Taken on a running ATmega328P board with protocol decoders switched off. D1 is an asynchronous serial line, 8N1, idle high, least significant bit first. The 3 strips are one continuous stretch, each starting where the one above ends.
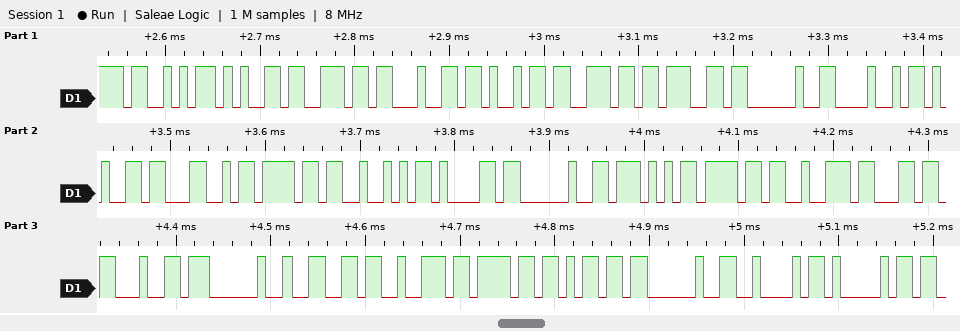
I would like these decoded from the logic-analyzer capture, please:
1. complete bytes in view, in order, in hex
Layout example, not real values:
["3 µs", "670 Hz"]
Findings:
["0x53 0x65 0x6E 0x64 0x69 0x6E 0x67 0x20 0x48 0x65 0x4C 0x6F 0x52 0x61 0x20 0x57 0x6F 0x72 0x6C 0x64 0x20 0x66 0x72 0x6F 0x6D 0x20 0x42 0x41"]
